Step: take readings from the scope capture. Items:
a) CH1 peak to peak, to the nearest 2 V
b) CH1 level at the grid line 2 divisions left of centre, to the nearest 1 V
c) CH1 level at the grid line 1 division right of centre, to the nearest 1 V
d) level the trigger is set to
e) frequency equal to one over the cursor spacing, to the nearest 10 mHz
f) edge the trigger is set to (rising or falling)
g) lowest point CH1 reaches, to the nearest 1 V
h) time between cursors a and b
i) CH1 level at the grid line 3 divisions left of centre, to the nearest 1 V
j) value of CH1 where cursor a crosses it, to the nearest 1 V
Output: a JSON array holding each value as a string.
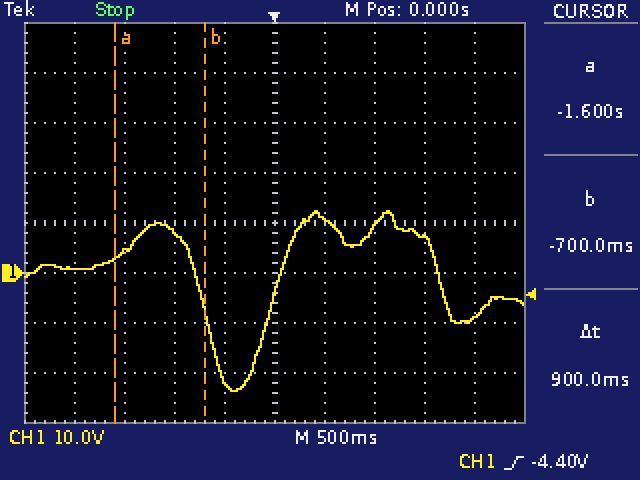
["36 V", "8 V", "11 V", "-4.40 V", "1.11 Hz", "rising", "-24 V", "900 ms", "4 V", "3 V"]
